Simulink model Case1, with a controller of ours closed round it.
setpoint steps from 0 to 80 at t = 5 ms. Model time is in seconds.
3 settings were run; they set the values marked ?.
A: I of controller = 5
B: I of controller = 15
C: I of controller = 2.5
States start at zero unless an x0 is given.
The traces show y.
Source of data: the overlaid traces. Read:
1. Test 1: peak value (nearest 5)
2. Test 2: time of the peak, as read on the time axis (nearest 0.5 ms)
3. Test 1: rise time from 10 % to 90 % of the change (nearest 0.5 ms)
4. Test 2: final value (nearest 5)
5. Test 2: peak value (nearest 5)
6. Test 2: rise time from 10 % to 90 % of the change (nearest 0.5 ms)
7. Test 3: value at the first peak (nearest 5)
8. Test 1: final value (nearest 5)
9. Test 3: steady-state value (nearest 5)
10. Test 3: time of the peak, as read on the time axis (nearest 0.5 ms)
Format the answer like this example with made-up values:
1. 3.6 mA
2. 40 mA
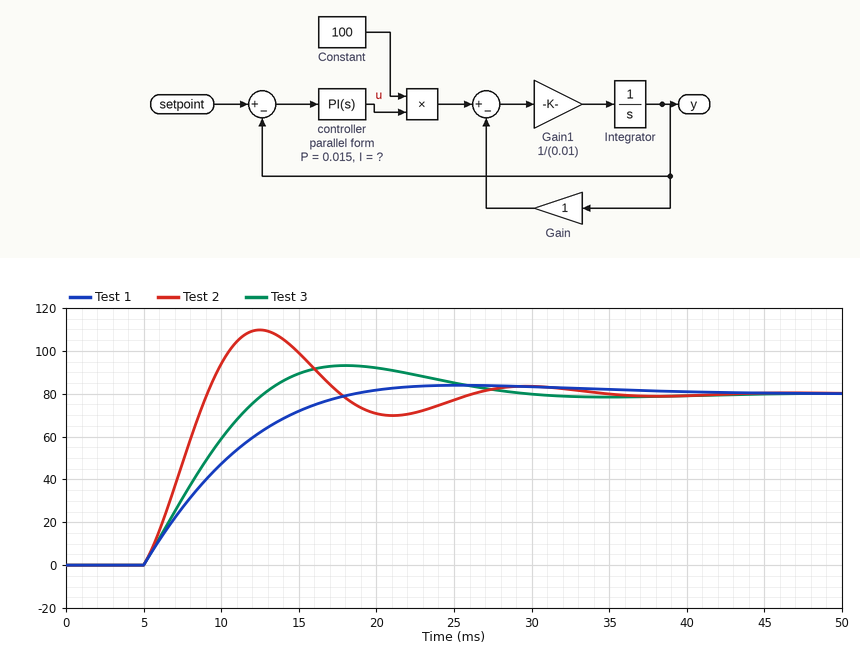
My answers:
1. 85
2. 12.5 ms
3. 9.5 ms
4. 80
5. 110
6. 3.0 ms
7. 95
8. 80
9. 80
10. 18.0 ms
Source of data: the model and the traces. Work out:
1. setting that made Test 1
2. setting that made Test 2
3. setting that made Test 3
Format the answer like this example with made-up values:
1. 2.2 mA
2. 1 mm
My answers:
1. C
2. B
3. A
